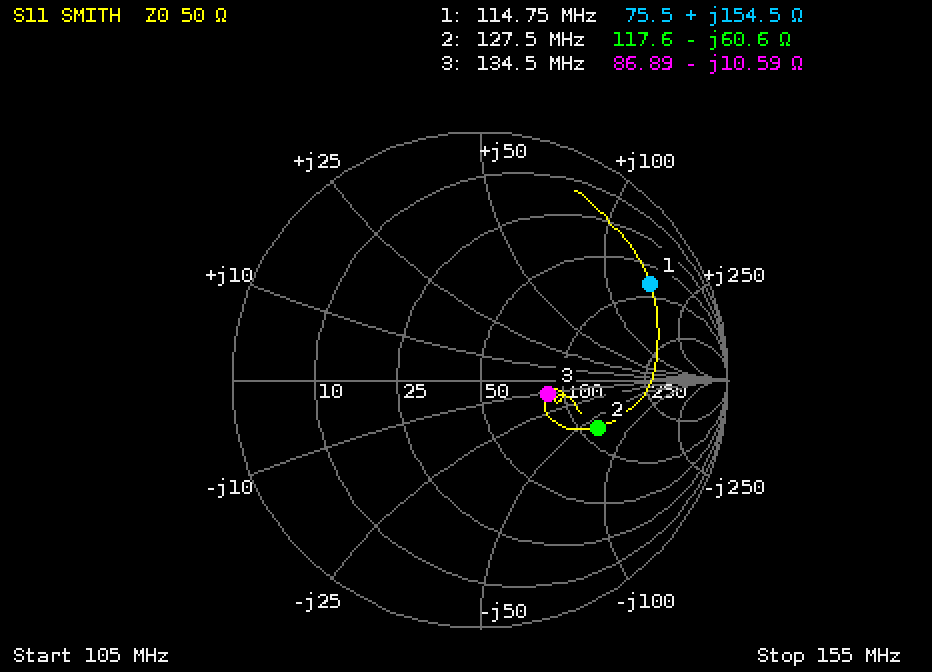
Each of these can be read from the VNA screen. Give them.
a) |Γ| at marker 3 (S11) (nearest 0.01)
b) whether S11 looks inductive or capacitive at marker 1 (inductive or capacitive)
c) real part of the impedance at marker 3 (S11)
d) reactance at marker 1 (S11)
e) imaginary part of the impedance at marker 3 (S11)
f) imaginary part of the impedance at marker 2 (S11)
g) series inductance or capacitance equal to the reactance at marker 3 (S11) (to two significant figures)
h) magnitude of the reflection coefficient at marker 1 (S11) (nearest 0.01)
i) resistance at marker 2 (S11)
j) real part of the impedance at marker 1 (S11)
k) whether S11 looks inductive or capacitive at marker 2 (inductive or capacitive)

0.28
inductive
86.89 Ω
+154.5 Ω
-10.59 Ω
-60.6 Ω
110 pF
0.79
117.6 Ω
75.5 Ω
capacitive
